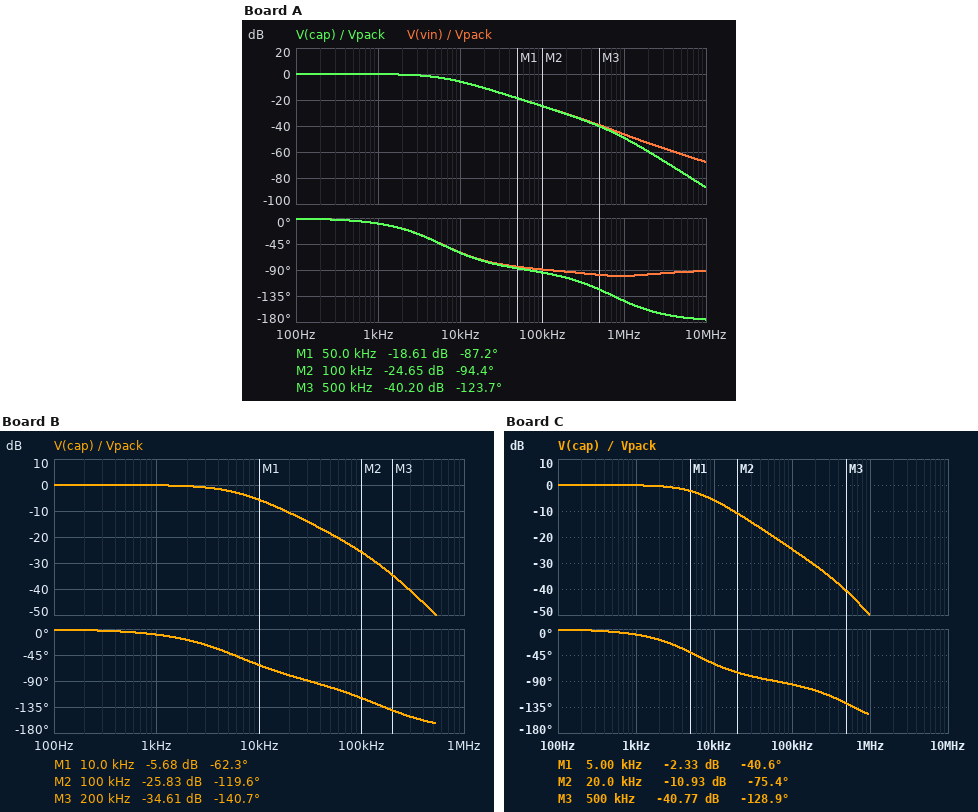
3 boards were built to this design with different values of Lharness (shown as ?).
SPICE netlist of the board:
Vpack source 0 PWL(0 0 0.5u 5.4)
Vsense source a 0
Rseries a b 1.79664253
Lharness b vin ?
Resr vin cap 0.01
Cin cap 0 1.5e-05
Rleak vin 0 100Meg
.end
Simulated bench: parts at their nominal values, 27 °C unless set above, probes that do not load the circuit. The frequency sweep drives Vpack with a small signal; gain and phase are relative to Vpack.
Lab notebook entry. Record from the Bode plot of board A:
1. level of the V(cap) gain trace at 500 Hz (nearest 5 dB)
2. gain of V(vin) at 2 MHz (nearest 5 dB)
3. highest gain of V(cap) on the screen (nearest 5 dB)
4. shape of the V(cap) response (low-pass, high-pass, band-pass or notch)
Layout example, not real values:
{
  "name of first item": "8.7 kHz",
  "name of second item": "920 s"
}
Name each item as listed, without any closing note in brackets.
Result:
{
  "level of the V(cap) gain trace at 500 Hz": "0 dB",
  "gain of V(vin) at 2 MHz": "-55 dB",
  "highest gain of V(cap) on the screen": "0 dB",
  "shape of the V(cap) response": "low-pass"
}
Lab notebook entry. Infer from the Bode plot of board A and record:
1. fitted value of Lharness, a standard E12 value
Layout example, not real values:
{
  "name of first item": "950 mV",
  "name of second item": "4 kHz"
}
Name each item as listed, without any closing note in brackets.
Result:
{
  "fitted value of Lharness, a standard E12 value": "390 nH"
}
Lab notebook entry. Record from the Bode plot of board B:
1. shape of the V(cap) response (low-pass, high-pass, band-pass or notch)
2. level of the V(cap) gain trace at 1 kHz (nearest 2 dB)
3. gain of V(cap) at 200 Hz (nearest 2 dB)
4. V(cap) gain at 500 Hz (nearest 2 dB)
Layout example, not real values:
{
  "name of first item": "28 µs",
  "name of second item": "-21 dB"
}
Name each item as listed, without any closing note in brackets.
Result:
{
  "shape of the V(cap) response": "low-pass",
  "level of the V(cap) gain trace at 1 kHz": "0 dB",
  "gain of V(cap) at 200 Hz": "0 dB",
  "V(cap) gain at 500 Hz": "0 dB"
}
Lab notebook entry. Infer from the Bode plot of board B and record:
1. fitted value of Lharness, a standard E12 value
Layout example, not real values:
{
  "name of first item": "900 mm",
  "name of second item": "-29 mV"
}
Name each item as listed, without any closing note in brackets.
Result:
{
  "fitted value of Lharness, a standard E12 value": "1.8 µH"
}
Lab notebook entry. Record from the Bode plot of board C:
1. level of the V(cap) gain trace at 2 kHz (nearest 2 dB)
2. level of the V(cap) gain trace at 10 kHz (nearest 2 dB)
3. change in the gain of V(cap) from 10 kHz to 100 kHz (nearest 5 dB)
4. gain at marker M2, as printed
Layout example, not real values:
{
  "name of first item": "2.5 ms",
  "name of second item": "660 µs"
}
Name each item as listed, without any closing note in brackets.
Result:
{
  "level of the V(cap) gain trace at 2 kHz": "0 dB",
  "level of the V(cap) gain trace at 10 kHz": "-6 dB",
  "change in the gain of V(cap) from 10 kHz to 100 kHz": "-20 dB",
  "gain at marker M2, as printed": "-10.93 dB"
}
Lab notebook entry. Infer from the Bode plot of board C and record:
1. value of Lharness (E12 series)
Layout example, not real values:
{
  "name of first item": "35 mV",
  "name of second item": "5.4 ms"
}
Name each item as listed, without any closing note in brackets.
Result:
{
  "value of Lharness": "470 nH"
}
